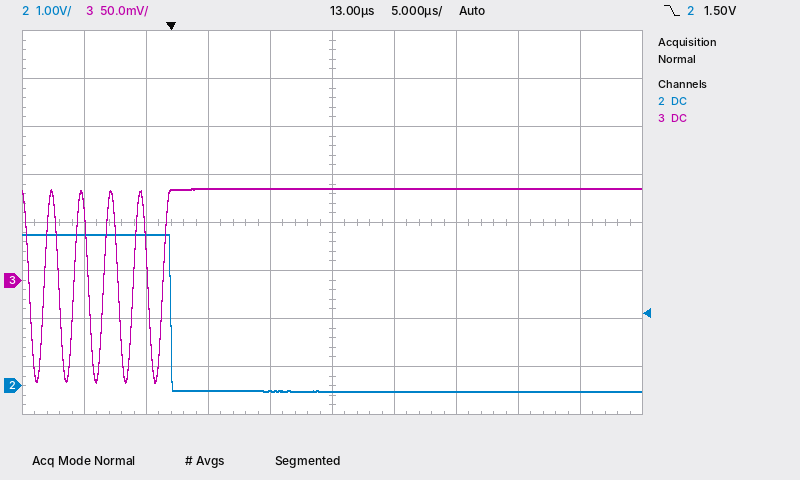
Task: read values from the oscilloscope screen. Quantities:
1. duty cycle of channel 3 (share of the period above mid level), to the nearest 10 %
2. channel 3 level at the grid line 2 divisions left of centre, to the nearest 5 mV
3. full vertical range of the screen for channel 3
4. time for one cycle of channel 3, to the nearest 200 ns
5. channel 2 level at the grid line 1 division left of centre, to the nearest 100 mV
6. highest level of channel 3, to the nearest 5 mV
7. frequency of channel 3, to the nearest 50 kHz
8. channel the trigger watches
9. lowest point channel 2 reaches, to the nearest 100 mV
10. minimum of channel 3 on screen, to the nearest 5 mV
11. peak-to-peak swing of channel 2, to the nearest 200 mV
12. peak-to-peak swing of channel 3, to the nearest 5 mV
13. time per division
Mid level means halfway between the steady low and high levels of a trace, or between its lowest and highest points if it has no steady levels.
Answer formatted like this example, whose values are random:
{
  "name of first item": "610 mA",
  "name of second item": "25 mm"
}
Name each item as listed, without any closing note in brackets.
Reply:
{
  "duty cycle of channel 3 (share of the period above mid level), to the nearest 10 %": "50 %",
  "channel 3 level at the grid line 2 divisions left of centre, to the nearest 5 mV": "95 mV",
  "full vertical range of the screen for channel 3": "400 mV",
  "time for one cycle of channel 3, to the nearest 200 ns": "2.4 µs",
  "channel 2 level at the grid line 1 division left of centre, to the nearest 100 mV": "-100 mV",
  "highest level of channel 3, to the nearest 5 mV": "95 mV",
  "frequency of channel 3, to the nearest 50 kHz": "400 kHz",
  "channel the trigger watches": "channel 2",
  "lowest point channel 2 reaches, to the nearest 100 mV": "-100 mV",
  "minimum of channel 3 on screen, to the nearest 5 mV": "-105 mV",
  "peak-to-peak swing of channel 2, to the nearest 200 mV": "3.2 V",
  "peak-to-peak swing of channel 3, to the nearest 5 mV": "200 mV",
  "time per division": "5 µs"
}
